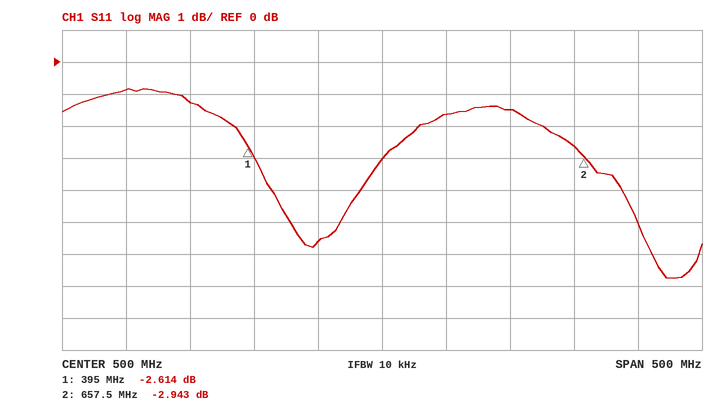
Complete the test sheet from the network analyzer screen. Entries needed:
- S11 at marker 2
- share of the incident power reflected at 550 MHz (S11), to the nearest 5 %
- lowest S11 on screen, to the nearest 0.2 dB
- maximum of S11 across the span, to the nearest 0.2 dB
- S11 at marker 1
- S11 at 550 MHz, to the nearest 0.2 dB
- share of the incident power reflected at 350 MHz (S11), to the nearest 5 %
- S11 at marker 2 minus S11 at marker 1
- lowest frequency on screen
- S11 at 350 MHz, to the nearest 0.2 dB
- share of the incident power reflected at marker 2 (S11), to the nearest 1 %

-2.943 dB
70 %
-6.8 dB
-0.8 dB
-2.614 dB
-1.6 dB
75 %
-0.329 dB
250 MHz
-1.2 dB
51 %
